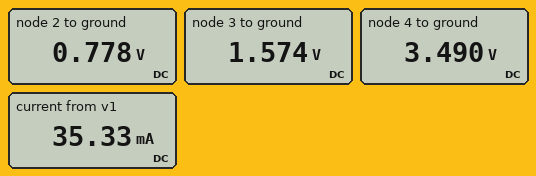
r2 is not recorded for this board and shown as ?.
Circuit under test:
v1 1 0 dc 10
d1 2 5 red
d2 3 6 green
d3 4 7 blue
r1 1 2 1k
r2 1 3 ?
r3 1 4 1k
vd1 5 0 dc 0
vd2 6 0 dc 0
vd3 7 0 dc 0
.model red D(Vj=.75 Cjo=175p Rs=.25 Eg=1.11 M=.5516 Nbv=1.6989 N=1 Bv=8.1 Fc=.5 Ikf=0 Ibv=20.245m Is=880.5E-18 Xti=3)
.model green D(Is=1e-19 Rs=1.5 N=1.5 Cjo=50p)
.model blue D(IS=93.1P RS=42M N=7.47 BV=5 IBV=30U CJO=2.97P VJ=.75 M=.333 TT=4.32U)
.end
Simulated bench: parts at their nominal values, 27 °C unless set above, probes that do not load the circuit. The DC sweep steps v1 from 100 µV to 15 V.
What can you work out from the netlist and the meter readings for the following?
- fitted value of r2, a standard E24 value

430 Ω
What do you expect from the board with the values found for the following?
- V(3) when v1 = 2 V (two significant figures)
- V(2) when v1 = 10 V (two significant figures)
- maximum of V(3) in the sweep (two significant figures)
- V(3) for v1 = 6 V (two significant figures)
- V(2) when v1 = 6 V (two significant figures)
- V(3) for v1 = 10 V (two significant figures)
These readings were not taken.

1.4 V
780 mV
1.6 V
1.5 V
760 mV
1.6 V
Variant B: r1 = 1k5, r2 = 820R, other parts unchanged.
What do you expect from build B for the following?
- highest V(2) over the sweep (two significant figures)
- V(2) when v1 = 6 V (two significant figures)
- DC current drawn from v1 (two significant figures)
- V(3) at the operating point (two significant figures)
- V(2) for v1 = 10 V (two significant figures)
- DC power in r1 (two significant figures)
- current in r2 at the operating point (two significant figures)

780 mV
750 mV
23 mA
1.5 V
770 mV
57 mW
10 mA
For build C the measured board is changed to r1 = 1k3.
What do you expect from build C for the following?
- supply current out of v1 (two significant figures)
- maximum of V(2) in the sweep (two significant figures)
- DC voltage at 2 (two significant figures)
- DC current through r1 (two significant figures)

33 mA
780 mV
770 mV
7.1 mA
